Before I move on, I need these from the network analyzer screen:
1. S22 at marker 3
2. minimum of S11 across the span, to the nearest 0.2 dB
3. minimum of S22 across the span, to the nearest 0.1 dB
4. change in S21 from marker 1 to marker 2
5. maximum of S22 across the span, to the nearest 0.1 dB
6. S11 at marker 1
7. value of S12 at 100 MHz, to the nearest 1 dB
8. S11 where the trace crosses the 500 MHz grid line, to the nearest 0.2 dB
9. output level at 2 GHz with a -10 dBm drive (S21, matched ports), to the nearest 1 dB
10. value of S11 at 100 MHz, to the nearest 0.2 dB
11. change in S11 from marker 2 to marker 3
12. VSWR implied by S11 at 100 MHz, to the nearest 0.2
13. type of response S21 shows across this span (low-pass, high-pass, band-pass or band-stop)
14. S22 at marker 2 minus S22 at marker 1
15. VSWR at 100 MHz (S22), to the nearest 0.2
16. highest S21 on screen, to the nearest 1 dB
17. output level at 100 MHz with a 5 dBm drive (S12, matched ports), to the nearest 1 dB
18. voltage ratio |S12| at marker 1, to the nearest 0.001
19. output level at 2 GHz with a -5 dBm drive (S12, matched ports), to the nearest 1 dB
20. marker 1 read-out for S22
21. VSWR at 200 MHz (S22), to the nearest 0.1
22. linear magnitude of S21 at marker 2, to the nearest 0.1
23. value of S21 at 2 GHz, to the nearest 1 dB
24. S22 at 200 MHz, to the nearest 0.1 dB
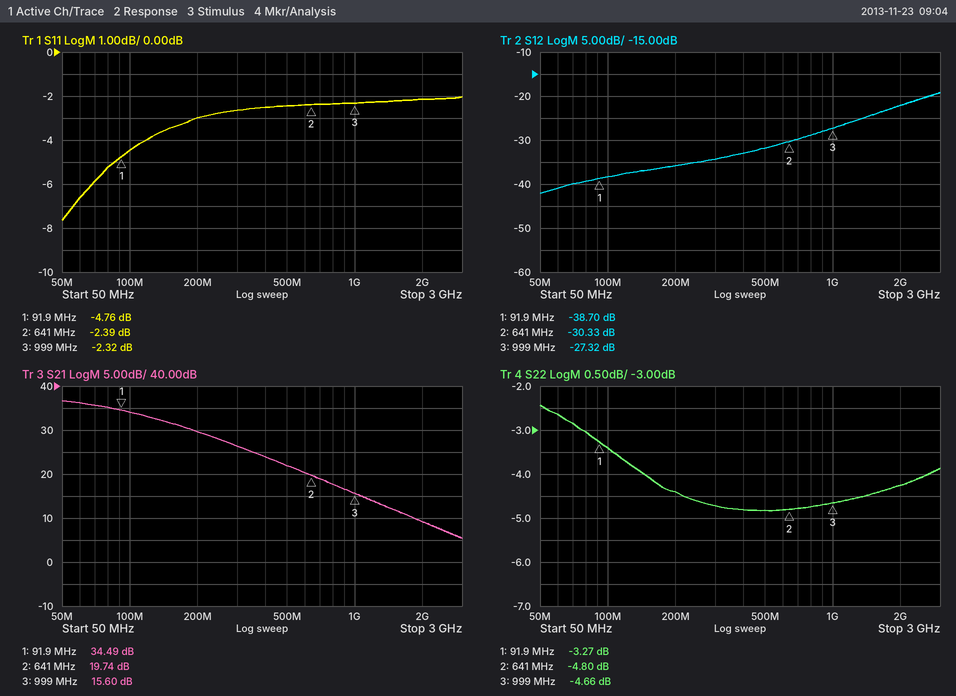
-4.66 dB
-7.6 dB
-4.8 dB
-14.75 dB
-2.4 dB
-4.76 dB
-38 dB
-2.4 dB
-1 dBm
-4.4 dB
0.07 dB
4.0
low-pass
-1.53 dB
5.2
37 dB
-33 dBm
0.012
-27 dBm
-3.27 dB
4.0
9.7
9 dB
-4.4 dB
